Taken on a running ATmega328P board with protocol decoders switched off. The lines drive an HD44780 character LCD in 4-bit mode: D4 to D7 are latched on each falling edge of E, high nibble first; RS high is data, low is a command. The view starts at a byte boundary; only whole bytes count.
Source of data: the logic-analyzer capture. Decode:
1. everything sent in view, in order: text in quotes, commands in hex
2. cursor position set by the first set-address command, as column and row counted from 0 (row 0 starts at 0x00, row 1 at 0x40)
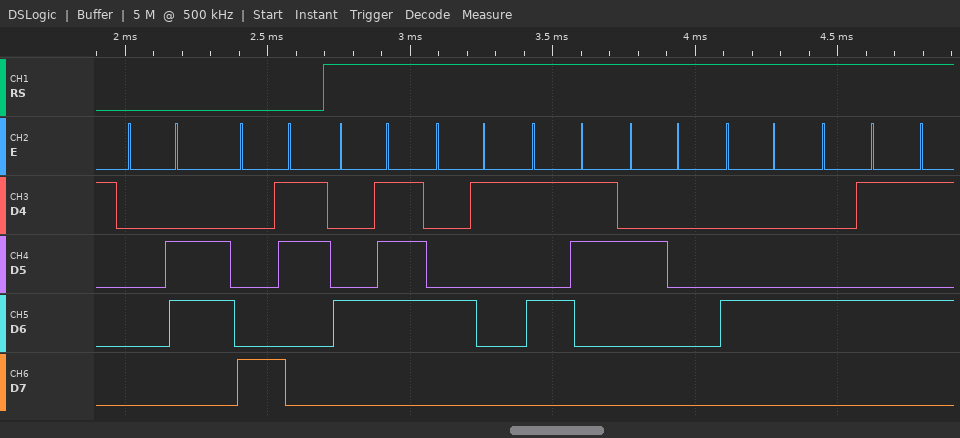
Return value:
0x06 0x83 "GAS DE"
column 3, row 0
